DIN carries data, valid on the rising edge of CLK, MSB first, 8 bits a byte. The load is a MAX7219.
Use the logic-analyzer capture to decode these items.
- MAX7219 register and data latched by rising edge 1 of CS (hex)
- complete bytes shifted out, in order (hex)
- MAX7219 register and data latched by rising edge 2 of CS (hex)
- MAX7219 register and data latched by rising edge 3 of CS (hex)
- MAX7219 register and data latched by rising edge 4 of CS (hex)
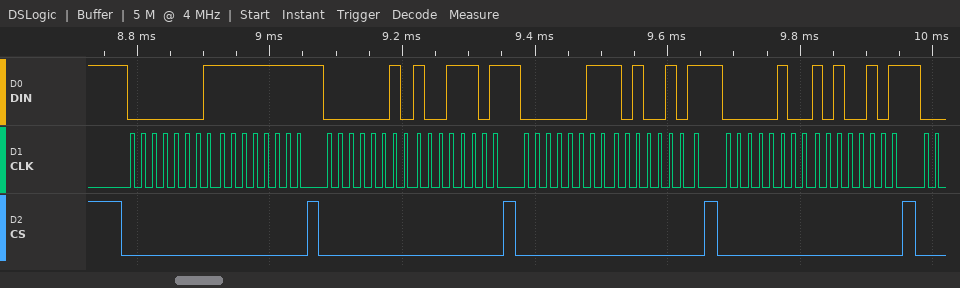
register 0x1, data 0xFF
01 FF 02 9D 03 A5 04 A5
register 0x2, data 0x9D
register 0x3, data 0xA5
register 0x4, data 0xA5
